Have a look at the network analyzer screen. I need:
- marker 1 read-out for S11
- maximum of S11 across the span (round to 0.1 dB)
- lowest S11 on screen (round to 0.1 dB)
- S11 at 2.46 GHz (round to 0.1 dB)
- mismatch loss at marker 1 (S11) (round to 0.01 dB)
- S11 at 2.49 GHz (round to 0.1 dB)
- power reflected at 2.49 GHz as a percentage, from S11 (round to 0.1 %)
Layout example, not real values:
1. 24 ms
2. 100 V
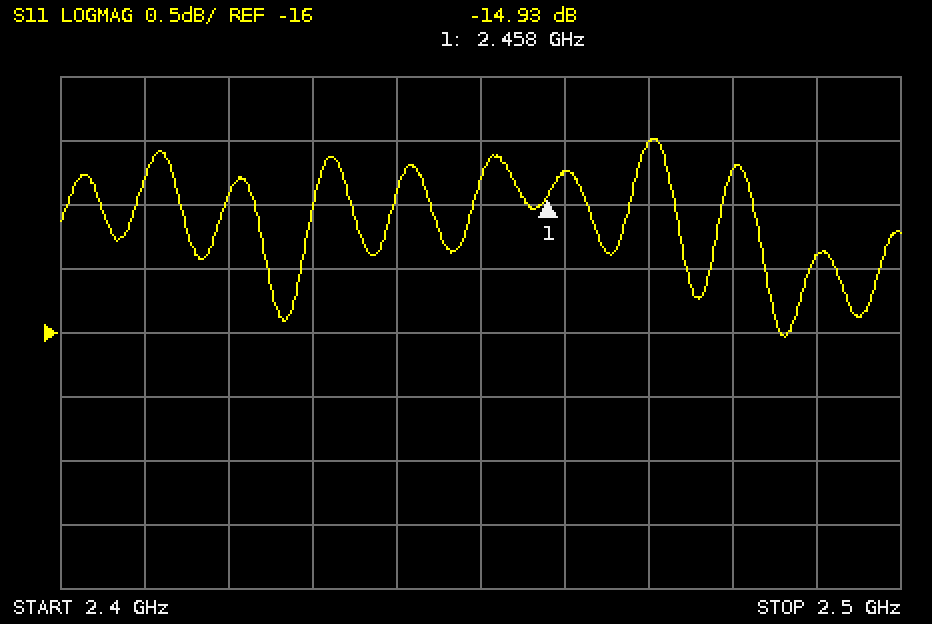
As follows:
1. -14.93 dB
2. -14.5 dB
3. -16.0 dB
4. -14.7 dB
5. 0.14 dB
6. -15.4 dB
7. 2.9 %
